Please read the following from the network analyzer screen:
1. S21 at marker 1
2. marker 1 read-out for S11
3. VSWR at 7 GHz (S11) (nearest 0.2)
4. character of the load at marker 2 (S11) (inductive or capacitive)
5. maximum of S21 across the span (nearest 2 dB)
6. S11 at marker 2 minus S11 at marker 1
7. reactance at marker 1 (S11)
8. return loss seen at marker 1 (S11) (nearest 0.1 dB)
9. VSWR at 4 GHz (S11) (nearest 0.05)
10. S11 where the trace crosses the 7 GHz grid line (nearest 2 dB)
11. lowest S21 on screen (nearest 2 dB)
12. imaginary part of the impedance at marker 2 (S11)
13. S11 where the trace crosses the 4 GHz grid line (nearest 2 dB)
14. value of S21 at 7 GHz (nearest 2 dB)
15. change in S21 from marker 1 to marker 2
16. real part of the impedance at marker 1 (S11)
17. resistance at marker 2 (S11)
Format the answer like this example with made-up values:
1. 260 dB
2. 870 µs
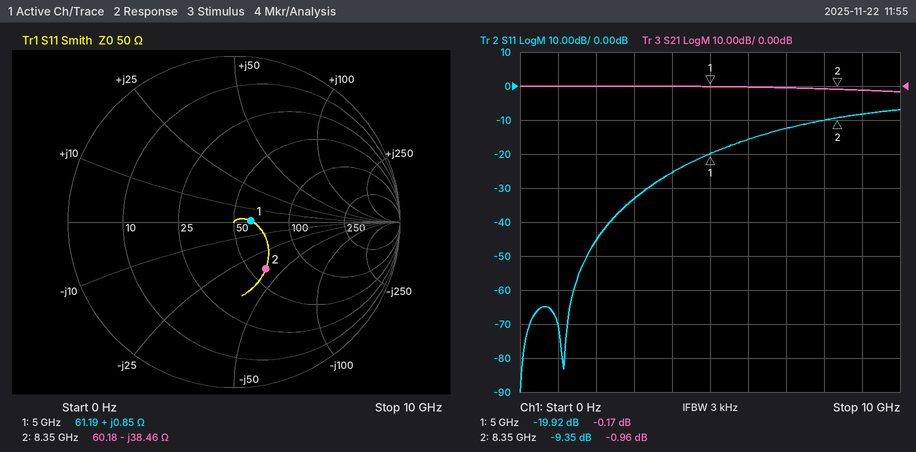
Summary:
1. -0.17 dB
2. -19.92 dB
3. 1.6
4. capacitive
5. 0 dB
6. 10.57 dB
7. +0.85 Ω
8. 19.9 dB
9. 1.10
10. -12 dB
11. -2 dB
12. -38.46 Ω
13. -26 dB
14. 0 dB
15. -0.79 dB
16. 61.19 Ω
17. 60.18 Ω
